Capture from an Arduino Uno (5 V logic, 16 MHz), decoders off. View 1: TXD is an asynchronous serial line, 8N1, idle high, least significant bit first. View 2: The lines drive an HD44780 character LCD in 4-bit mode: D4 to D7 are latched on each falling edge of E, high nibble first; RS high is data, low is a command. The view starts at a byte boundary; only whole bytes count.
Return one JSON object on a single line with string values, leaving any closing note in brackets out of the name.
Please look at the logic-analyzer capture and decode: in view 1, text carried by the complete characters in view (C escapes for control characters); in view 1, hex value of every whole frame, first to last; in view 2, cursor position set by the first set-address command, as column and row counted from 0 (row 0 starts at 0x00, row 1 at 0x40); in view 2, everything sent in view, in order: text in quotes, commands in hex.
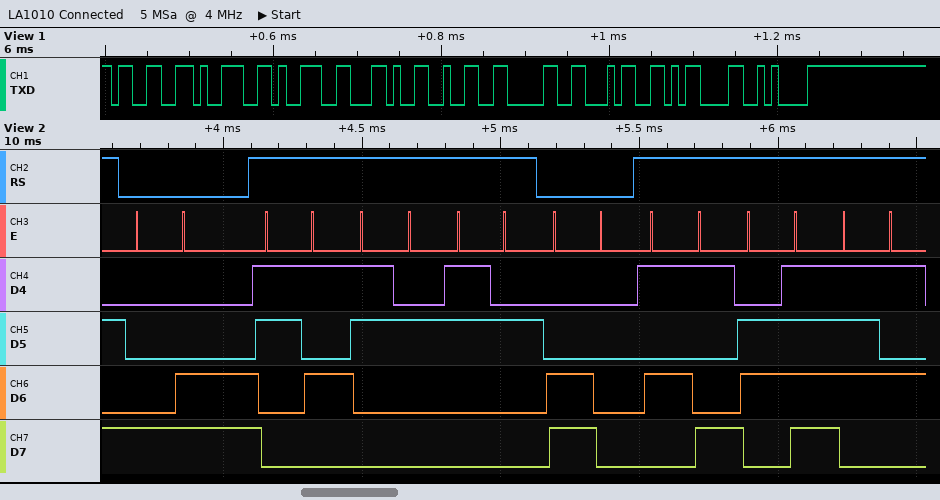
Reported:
{"in view 1, text carried by the complete characters in view": "\"399,204\\r\\n\"", "in view 1, hex value of every whole frame, first to last": "33 39 39 2C 32 30 34 0D 0A", "in view 2, cursor position set by the first set-address command, as column and row counted from 0": "column 12, row 0", "in view 2, everything sent in view, in order: text in quotes, commands in hex": "0x8C \"522\" 0xC0 \"You\""}
